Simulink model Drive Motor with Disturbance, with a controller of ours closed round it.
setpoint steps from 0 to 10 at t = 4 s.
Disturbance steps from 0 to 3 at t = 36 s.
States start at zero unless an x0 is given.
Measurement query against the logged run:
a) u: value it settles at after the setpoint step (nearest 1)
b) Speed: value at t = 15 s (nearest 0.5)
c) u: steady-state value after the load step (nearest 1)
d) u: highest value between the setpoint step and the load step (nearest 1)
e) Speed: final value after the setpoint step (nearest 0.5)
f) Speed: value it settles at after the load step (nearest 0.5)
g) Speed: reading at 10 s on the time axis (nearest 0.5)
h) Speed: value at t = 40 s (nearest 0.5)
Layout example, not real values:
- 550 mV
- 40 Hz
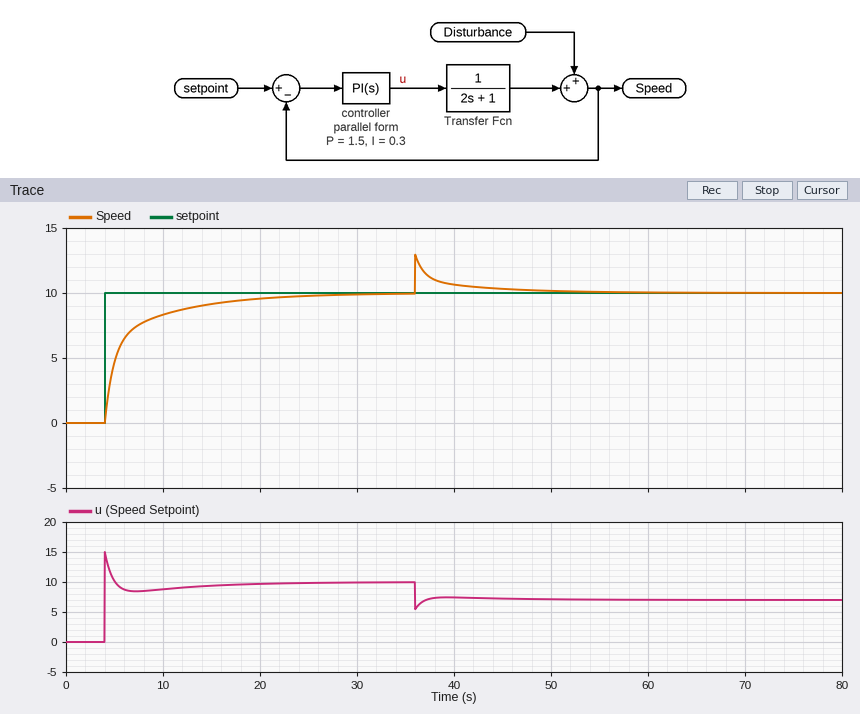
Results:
- 10
- 9.0
- 7
- 15
- 10.0
- 10.0
- 8.5
- 10.5
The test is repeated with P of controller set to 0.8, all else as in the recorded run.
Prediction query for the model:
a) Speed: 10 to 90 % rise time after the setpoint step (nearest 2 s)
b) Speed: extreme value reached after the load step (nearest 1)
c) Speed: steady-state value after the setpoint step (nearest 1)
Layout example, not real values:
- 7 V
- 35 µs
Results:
- 8 s
- 13
- 10
